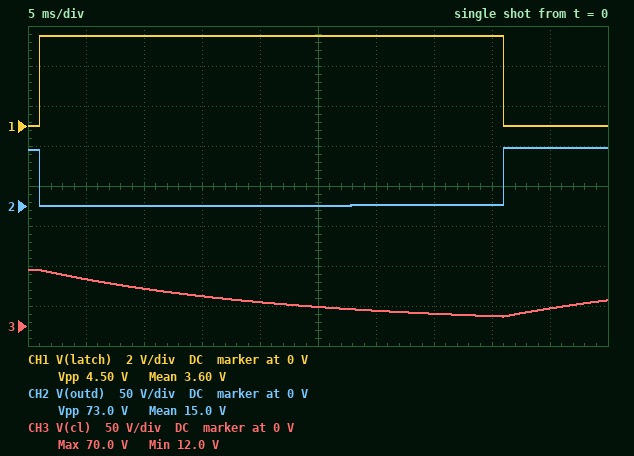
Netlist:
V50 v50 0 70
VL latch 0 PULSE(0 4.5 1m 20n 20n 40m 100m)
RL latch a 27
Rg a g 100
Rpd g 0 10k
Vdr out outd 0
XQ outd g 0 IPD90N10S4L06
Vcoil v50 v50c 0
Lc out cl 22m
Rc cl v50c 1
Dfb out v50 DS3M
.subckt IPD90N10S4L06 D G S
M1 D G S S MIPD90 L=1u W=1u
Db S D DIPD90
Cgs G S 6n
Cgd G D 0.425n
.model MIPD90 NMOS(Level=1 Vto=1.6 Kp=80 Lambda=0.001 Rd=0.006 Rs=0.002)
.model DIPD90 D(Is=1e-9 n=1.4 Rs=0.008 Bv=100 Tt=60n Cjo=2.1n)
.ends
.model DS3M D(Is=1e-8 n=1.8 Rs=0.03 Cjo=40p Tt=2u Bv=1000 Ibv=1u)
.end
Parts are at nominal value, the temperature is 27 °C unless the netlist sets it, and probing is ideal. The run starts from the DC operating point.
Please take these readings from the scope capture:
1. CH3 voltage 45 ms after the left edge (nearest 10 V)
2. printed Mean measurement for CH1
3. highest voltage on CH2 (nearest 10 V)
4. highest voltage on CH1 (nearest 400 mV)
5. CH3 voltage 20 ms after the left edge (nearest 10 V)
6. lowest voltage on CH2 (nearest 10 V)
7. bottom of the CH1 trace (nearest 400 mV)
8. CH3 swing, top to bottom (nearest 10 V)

20 V
3.60 V
70 V
4.4 V
30 V
0 V
0 V
60 V
